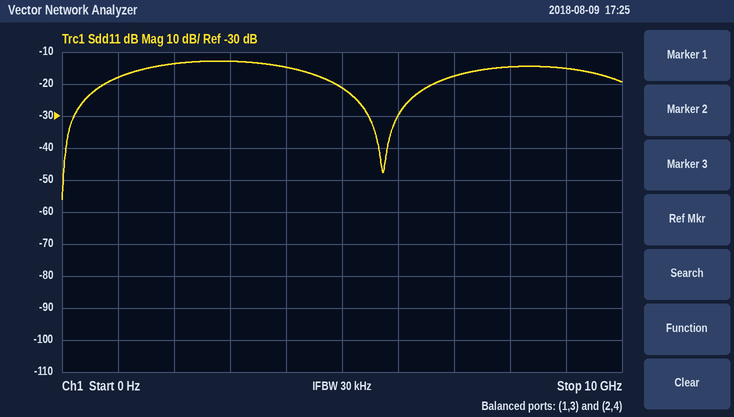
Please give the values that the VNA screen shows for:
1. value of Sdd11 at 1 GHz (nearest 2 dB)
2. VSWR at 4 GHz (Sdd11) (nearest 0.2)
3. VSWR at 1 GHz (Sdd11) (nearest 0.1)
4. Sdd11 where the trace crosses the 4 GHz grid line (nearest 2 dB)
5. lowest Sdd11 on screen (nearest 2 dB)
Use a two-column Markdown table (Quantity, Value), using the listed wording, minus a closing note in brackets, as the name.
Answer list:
| Quantity | Value |
|---|---|
| value of Sdd11 at 1 GHz | -18 dB |
| VSWR at 4 GHz (Sdd11) | 1.4 |
| VSWR at 1 GHz (Sdd11) | 1.3 |
| Sdd11 where the trace crosses the 4 GHz grid line | -14 dB |
| lowest Sdd11 on screen | -56 dB |
